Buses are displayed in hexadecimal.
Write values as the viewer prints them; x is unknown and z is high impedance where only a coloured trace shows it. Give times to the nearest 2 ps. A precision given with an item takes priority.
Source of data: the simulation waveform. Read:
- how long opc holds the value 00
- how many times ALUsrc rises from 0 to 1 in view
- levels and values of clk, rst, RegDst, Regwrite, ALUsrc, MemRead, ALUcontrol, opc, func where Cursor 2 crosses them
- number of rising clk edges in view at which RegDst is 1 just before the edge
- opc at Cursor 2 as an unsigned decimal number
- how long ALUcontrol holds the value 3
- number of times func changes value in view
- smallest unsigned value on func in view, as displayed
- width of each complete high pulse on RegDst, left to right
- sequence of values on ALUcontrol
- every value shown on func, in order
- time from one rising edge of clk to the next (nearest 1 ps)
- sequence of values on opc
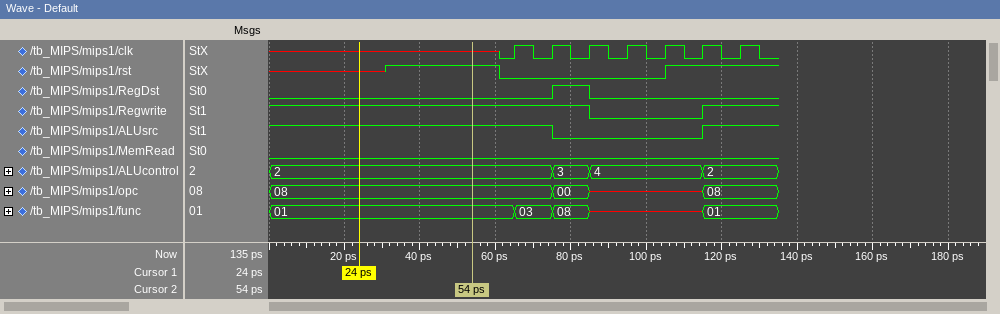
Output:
10 ps
1
clk=x, rst=1, RegDst=0, Regwrite=1, ALUsrc=1, MemRead=0, ALUcontrol=2, opc=08, func=01
1
8
10 ps
4
01
10 ps
2, 3, 4, 2
01, 03, 08, x, 01
10 ps
08, 00, x, 08
